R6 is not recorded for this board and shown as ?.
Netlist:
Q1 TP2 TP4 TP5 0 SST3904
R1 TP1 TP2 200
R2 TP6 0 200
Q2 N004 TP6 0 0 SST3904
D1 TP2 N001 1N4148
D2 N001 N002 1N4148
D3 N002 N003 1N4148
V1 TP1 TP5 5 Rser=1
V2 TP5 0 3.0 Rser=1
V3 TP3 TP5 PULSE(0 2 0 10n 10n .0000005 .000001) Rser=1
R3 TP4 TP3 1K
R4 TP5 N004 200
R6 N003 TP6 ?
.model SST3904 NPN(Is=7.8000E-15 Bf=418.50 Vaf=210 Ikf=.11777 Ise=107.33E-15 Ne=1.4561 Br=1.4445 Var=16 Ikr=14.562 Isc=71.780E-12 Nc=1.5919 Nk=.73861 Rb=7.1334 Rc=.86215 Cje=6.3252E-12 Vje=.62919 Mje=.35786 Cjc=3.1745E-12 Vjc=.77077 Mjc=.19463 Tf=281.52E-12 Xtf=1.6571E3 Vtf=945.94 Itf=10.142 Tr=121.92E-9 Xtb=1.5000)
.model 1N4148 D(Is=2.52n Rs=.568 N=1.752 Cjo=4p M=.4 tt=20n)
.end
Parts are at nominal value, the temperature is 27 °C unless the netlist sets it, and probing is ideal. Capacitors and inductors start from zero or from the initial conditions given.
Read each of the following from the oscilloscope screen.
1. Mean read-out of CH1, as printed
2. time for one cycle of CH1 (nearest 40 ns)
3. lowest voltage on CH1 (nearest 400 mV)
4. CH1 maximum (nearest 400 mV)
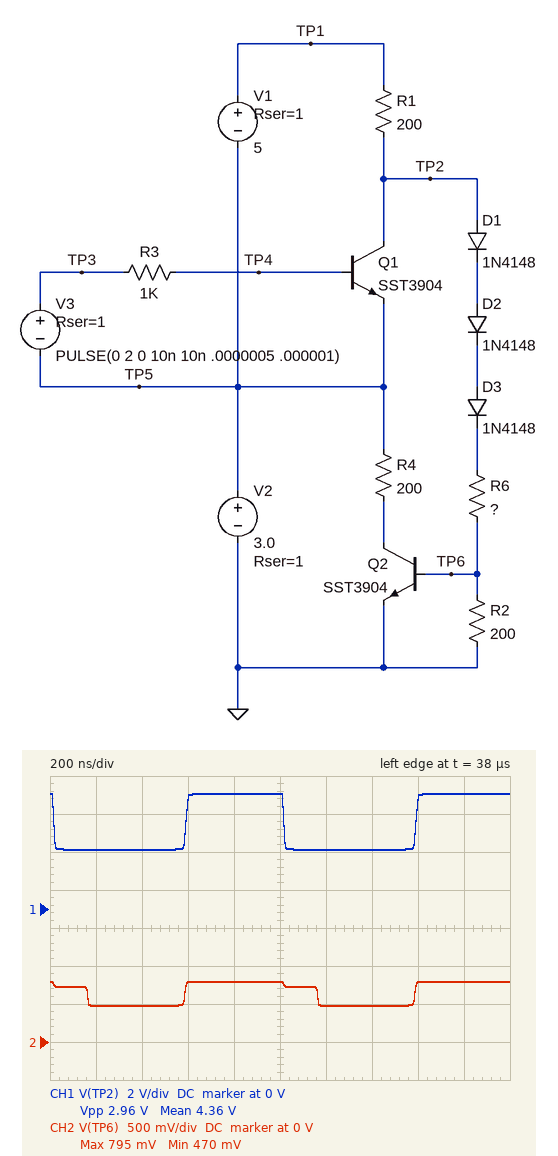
4.36 V
1.00 µs
3.2 V
6.0 V
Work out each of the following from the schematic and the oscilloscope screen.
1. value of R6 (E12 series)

330 Ω
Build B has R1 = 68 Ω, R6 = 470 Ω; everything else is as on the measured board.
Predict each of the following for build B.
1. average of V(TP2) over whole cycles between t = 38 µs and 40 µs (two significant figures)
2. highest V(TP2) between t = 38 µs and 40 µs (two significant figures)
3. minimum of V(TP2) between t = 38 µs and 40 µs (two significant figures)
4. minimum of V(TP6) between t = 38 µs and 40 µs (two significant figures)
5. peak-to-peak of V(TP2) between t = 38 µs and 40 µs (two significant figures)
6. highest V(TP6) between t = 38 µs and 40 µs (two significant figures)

5.1 V
7.3 V
3.2 V
410 mV
4.1 V
790 mV
